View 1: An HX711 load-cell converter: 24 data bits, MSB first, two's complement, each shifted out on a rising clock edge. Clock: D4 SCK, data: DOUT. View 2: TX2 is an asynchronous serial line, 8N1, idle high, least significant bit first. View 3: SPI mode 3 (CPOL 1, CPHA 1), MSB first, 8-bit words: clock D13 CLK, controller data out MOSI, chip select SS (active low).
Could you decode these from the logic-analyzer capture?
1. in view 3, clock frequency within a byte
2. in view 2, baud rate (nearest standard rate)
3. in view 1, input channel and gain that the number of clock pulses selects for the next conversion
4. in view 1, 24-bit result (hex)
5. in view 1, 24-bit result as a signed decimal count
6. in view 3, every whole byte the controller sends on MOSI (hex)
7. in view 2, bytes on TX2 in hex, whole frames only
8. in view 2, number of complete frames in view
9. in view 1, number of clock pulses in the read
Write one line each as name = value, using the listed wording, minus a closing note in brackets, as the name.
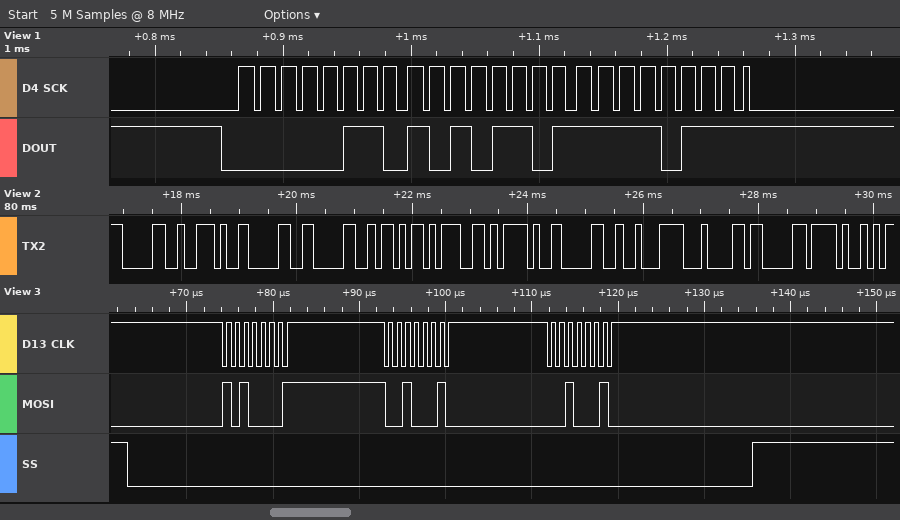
in view 3, clock frequency within a byte = 1 MHz
in view 2, baud rate = 9600 baud
in view 1, input channel and gain that the number of clock pulses selects for the next conversion = channel A, gain 128
in view 1, 24-bit result = 0x06ADF7
in view 1, 24-bit result as a signed decimal count = 437751
in view 3, every whole byte the controller sends on MOSI = 0xA1 0x22 0x22
in view 2, bytes on TX2 in hex, whole frames only = 30 2E 30 30 6B 67 2F 30 E2 84 83 2F
in view 2, number of complete frames in view = 12
in view 1, number of clock pulses in the read = 25
